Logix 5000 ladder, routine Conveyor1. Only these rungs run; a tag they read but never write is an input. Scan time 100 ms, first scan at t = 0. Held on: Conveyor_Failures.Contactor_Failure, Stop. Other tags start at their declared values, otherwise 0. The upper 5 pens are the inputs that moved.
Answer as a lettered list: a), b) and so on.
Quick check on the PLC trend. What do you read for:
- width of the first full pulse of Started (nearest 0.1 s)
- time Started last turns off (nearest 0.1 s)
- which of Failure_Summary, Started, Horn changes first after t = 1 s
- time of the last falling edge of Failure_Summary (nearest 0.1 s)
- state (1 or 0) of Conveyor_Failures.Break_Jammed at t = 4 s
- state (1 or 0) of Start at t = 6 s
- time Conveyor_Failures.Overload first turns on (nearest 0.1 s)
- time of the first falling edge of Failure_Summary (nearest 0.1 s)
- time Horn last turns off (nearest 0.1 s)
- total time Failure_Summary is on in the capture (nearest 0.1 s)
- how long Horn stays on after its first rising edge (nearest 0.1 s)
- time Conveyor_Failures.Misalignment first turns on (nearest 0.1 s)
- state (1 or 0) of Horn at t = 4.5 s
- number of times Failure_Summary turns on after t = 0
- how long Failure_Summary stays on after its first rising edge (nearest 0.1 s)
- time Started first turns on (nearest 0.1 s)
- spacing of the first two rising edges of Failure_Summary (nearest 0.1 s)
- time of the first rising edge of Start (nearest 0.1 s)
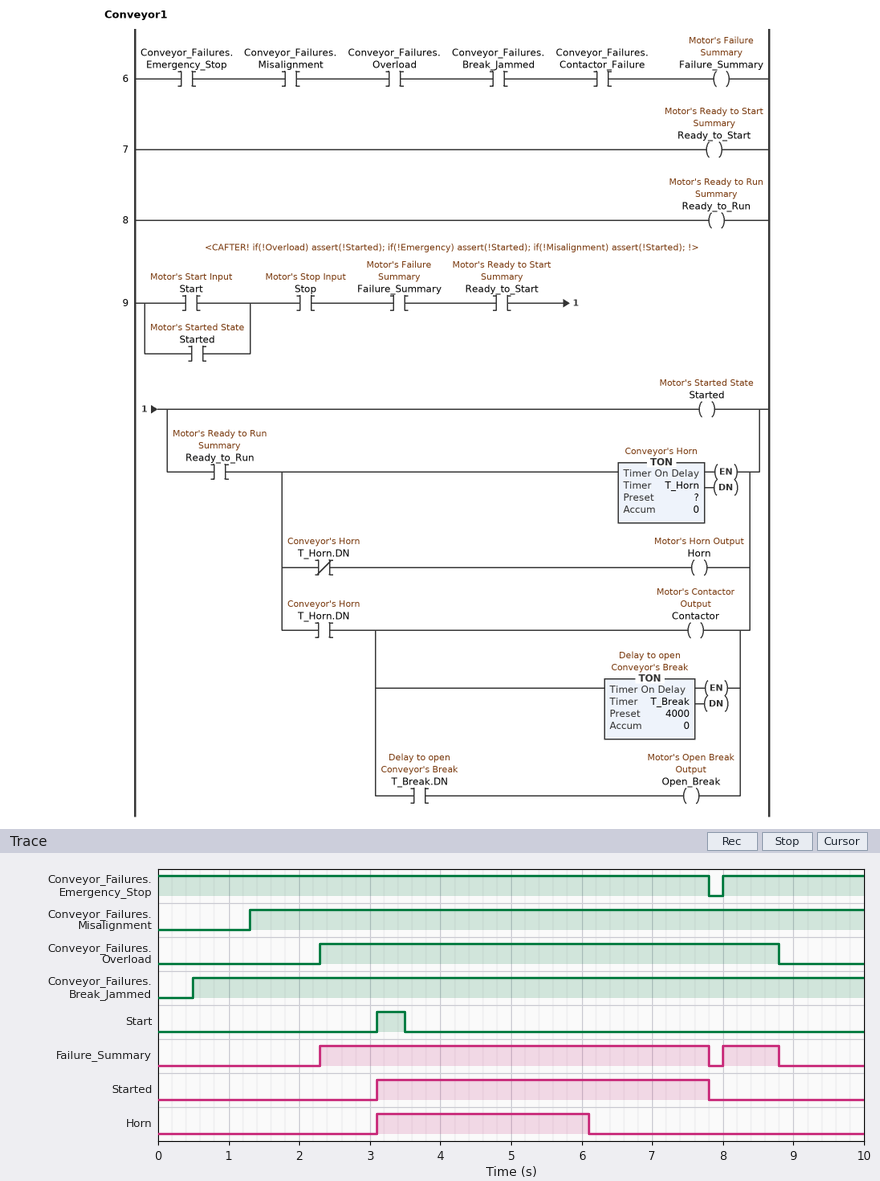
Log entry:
a) 4.7 s
b) 7.8 s
c) Failure_Summary
d) 8.8 s
e) 1
f) 0
g) 2.3 s
h) 7.8 s
i) 6.1 s
j) 6.3 s
k) 3.0 s
l) 1.3 s
m) 1
n) 2
o) 5.5 s
p) 3.1 s
q) 5.7 s
r) 3.1 s
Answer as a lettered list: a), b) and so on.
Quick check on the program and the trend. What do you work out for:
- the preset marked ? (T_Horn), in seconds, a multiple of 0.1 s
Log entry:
a) 3.0 s
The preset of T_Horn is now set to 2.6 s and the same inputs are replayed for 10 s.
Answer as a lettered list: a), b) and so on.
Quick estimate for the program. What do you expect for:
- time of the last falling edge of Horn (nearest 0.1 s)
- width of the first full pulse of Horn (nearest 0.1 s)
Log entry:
a) 5.7 s
b) 2.6 s
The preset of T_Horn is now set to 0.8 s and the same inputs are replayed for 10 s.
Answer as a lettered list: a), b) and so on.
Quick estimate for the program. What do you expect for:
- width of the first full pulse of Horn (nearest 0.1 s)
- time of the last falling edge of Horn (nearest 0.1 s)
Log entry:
a) 0.8 s
b) 3.9 s
